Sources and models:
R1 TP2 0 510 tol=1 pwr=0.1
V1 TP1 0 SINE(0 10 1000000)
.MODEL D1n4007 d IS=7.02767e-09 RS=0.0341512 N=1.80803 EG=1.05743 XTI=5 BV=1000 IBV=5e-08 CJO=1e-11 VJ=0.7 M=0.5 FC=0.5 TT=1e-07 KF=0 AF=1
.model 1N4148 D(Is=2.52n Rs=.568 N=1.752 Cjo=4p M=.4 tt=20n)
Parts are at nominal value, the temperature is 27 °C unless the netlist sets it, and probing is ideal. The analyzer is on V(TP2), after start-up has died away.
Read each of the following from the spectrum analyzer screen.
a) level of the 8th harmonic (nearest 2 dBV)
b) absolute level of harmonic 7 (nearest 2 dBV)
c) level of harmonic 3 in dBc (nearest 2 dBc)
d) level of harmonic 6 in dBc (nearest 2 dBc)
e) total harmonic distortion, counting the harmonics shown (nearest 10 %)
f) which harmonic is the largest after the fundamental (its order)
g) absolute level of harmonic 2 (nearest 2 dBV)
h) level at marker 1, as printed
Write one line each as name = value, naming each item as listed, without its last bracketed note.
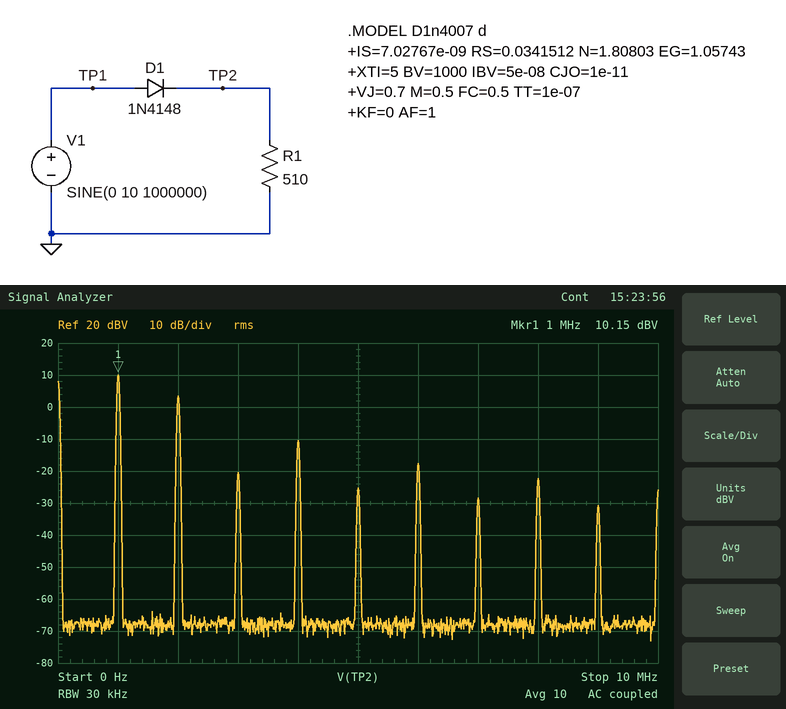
level of the 8th harmonic = -22 dBV
absolute level of harmonic 7 = -28 dBV
level of harmonic 3 in dBc = -30 dBc
level of harmonic 6 in dBc = -28 dBc
total harmonic distortion, counting the harmonics shown = 50 %
which harmonic is the largest after the fundamental = 2
absolute level of harmonic 2 = 4 dBV
level at marker 1, as printed = 10.15 dBV
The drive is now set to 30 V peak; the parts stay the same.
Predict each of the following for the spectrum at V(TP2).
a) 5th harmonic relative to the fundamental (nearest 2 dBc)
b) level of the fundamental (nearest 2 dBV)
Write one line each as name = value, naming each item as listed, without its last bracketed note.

5th harmonic relative to the fundamental = -42 dBc
level of the fundamental = 20 dBV
